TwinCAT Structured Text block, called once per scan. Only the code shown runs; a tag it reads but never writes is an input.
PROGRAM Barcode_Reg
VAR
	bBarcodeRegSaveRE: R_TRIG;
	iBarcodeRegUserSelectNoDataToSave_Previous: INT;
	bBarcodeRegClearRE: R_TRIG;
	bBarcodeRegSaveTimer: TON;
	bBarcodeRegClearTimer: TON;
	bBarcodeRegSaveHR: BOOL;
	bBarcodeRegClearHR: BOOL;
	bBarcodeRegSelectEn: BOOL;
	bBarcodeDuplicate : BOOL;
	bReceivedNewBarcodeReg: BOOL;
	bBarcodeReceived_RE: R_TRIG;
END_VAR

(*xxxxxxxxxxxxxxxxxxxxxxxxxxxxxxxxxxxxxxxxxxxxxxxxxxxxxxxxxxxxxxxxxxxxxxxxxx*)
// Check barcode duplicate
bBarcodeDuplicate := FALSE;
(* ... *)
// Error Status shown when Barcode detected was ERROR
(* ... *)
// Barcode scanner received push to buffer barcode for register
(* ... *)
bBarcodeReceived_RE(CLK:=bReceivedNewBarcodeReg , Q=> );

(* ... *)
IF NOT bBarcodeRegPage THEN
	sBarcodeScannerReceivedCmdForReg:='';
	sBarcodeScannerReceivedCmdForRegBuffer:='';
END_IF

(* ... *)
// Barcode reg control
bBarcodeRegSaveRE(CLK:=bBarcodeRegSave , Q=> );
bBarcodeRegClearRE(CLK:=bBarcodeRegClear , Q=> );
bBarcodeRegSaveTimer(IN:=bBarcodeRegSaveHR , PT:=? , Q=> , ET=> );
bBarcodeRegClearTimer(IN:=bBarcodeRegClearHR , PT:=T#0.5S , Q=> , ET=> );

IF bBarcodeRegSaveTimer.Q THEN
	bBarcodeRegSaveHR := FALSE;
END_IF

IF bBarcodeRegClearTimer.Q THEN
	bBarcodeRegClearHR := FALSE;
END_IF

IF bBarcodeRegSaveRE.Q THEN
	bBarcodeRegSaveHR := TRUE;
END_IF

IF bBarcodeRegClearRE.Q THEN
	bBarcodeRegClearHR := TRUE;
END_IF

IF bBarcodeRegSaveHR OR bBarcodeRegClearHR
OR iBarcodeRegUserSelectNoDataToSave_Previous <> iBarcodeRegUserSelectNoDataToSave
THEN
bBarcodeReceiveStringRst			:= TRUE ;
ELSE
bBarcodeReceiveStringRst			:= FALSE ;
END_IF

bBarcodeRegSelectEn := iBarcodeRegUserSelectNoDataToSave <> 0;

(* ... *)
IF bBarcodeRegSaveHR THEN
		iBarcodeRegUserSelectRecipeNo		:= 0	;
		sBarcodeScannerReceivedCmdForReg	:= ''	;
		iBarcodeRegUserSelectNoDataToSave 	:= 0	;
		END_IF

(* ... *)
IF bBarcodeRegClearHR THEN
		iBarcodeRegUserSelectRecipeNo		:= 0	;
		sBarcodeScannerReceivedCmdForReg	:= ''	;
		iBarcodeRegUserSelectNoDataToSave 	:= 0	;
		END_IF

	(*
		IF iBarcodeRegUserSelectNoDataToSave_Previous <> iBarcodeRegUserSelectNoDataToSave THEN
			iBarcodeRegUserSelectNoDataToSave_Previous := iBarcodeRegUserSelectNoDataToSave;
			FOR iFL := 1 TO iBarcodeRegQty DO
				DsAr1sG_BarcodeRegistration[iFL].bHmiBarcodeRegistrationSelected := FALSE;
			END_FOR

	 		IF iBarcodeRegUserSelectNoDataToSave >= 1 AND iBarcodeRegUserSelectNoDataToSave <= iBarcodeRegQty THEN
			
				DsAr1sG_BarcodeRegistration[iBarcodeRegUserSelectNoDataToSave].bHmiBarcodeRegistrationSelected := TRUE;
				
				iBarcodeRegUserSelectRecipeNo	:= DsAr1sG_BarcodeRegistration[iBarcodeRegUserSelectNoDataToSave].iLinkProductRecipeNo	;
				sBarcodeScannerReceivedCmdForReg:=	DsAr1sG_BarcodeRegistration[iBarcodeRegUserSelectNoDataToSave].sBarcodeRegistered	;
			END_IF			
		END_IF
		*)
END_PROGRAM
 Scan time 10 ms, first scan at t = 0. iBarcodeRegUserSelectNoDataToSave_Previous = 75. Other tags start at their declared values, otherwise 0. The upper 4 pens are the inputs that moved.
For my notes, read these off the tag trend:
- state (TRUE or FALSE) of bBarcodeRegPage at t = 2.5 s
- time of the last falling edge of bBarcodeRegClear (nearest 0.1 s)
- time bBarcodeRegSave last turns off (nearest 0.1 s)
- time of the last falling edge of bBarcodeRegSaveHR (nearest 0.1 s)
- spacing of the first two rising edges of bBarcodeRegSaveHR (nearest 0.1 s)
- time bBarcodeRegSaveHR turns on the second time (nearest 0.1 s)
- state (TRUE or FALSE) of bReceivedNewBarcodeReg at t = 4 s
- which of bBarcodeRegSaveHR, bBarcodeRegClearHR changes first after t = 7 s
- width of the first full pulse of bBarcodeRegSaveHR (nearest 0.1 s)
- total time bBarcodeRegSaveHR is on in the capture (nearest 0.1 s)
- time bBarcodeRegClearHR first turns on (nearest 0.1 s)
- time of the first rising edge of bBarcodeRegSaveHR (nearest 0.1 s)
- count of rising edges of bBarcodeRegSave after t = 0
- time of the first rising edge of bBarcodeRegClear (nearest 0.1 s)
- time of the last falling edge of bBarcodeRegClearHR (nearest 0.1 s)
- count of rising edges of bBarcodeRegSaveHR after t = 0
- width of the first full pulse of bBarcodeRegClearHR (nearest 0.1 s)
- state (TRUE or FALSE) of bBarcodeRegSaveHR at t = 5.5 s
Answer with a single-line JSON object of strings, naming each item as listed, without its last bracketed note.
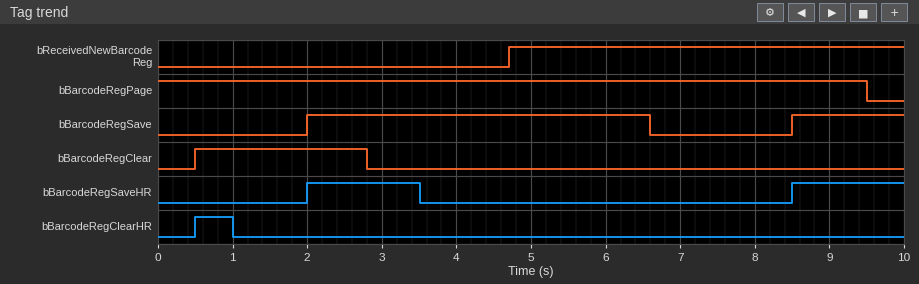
{"state (TRUE or FALSE) of bBarcodeRegPage at t = 2.5 s": "TRUE", "time of the last falling edge of bBarcodeRegClear": "2.8 s", "time bBarcodeRegSave last turns off": "6.6 s", "time of the last falling edge of bBarcodeRegSaveHR": "3.5 s", "spacing of the first two rising edges of bBarcodeRegSaveHR": "6.5 s", "time bBarcodeRegSaveHR turns on the second time": "8.5 s", "state (TRUE or FALSE) of bReceivedNewBarcodeReg at t = 4 s": "FALSE", "which of bBarcodeRegSaveHR, bBarcodeRegClearHR changes first after t = 7 s": "bBarcodeRegSaveHR", "width of the first full pulse of bBarcodeRegSaveHR": "1.5 s", "total time bBarcodeRegSaveHR is on in the capture": "3.0 s", "time bBarcodeRegClearHR first turns on": "0.5 s", "time of the first rising edge of bBarcodeRegSaveHR": "2.0 s", "count of rising edges of bBarcodeRegSave after t = 0": "2", "time of the first rising edge of bBarcodeRegClear": "0.5 s", "time of the last falling edge of bBarcodeRegClearHR": "1.0 s", "count of rising edges of bBarcodeRegSaveHR after t = 0": "2", "width of the first full pulse of bBarcodeRegClearHR": "0.5 s", "state (TRUE or FALSE) of bBarcodeRegSaveHR at t = 5.5 s": "FALSE"}
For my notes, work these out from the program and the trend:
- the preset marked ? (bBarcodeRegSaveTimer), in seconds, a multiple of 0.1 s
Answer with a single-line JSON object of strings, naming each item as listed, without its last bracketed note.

{"the preset marked ? (bBarcodeRegSaveTimer), in seconds, a multiple of 0.1 s": "1.5 s"}
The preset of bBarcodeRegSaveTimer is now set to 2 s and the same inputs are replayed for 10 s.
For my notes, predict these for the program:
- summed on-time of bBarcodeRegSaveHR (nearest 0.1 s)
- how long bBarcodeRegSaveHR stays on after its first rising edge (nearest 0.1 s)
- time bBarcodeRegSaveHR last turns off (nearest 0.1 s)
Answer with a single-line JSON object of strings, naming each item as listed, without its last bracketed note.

{"summed on-time of bBarcodeRegSaveHR": "3.5 s", "how long bBarcodeRegSaveHR stays on after its first rising edge": "2.0 s", "time bBarcodeRegSaveHR last turns off": "4.0 s"}
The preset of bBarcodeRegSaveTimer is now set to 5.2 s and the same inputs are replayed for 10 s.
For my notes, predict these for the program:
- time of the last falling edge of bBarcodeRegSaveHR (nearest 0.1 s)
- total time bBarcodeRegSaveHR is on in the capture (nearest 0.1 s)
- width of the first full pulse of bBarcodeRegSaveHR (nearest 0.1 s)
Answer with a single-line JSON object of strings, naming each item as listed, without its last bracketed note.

{"time of the last falling edge of bBarcodeRegSaveHR": "7.2 s", "total time bBarcodeRegSaveHR is on in the capture": "6.7 s", "width of the first full pulse of bBarcodeRegSaveHR": "5.2 s"}
